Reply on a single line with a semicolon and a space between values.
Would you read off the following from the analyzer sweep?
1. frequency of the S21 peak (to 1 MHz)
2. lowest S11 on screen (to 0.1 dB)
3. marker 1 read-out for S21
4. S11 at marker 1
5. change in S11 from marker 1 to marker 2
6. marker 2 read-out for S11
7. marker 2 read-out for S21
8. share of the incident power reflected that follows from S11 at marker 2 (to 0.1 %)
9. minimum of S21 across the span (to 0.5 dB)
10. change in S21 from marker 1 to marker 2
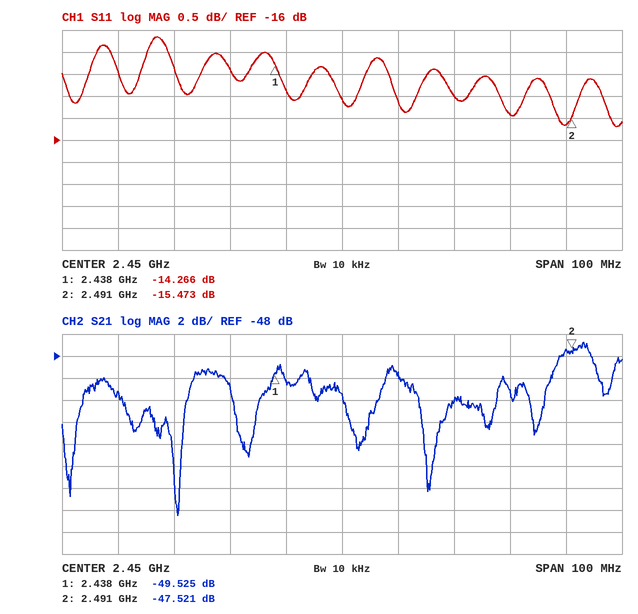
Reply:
2.493 GHz; -15.7 dB; -49.525 dB; -14.266 dB; -1.207 dB; -15.473 dB; -47.521 dB; 2.8 %; -62.5 dB; 2.004 dB
